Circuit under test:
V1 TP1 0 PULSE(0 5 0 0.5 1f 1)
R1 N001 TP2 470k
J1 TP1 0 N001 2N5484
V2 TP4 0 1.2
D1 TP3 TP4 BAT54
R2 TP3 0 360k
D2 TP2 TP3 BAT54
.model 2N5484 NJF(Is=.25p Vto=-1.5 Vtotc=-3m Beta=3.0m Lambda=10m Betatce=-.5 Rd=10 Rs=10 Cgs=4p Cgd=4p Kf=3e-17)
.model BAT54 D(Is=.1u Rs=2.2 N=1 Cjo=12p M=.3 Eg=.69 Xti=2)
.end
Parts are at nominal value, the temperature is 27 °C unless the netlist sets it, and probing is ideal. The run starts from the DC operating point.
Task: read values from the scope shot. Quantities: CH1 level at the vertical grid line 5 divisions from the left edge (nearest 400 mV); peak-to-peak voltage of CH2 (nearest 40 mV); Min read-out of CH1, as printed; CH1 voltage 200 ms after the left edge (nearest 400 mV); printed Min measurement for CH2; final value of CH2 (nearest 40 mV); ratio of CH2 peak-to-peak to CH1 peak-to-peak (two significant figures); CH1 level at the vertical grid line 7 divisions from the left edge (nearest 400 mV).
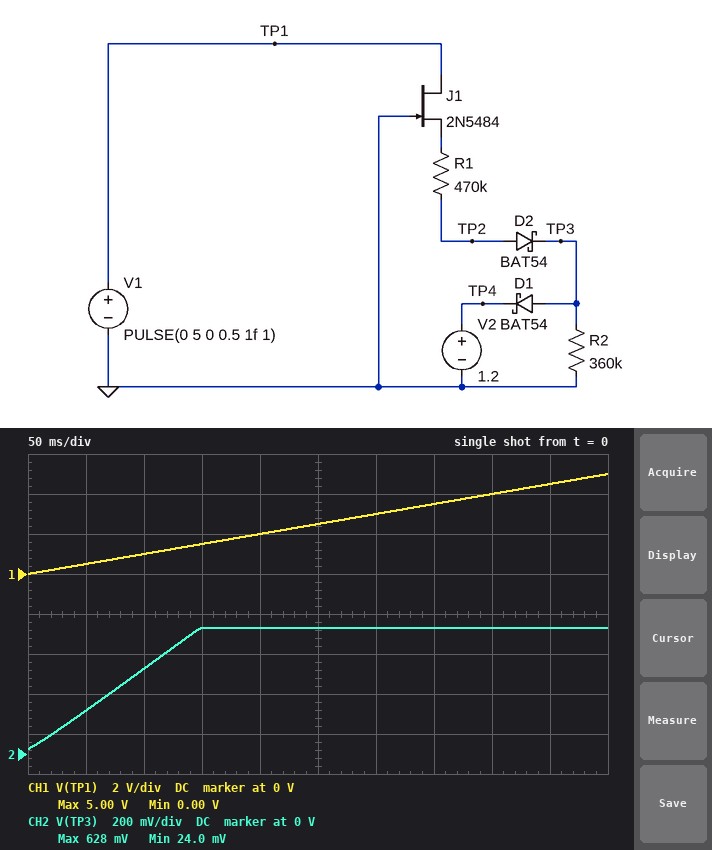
2.4 V
600 mV
0.00 V
2.0 V
24.0 mV
640 mV
0.12
3.6 V
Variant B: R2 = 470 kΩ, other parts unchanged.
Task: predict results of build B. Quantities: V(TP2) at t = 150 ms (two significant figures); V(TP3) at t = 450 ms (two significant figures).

800 mV
730 mV
